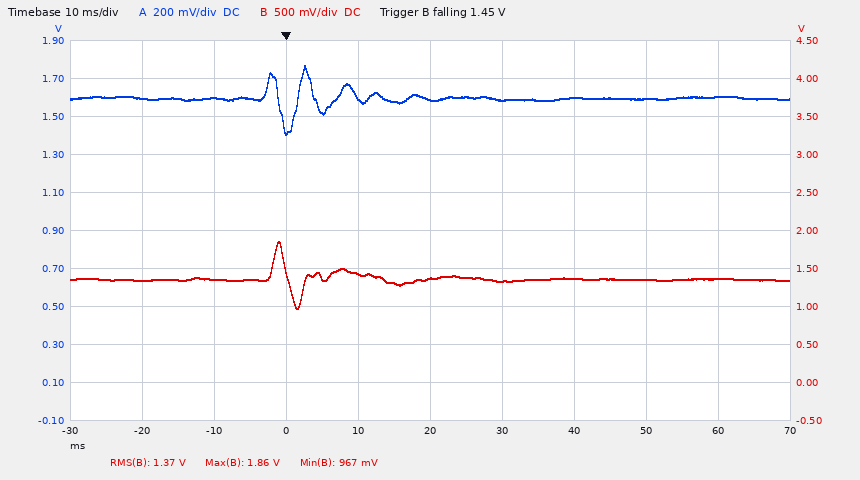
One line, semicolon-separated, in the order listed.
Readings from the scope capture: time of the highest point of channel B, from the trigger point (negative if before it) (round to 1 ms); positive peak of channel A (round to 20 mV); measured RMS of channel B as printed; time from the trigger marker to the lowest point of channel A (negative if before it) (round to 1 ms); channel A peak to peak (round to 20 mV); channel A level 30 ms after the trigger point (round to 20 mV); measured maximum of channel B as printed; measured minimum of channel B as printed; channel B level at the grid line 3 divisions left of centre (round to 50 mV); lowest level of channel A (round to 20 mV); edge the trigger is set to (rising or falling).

-1 ms; 1.76 V; 1.37 V; 0 ms; 360 mV; 1.58 V; 1.86 V; 967 mV; 1.35 V; 1.40 V; falling
